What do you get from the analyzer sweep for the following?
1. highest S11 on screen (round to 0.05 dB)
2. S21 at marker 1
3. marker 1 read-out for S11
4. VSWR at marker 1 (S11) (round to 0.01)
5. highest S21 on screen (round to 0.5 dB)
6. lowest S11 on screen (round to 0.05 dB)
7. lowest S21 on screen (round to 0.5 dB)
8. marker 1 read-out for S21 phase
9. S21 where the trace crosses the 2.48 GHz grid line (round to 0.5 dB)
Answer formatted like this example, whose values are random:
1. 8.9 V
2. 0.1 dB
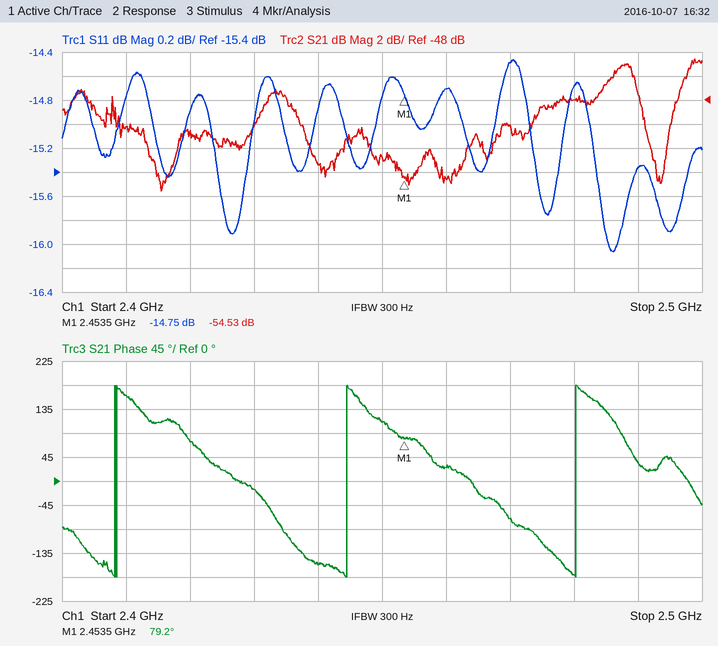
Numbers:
1. -14.45 dB
2. -54.53 dB
3. -14.75 dB
4. 1.45
5. -44.5 dB
6. -16.05 dB
7. -55.5 dB
8. 79.2°
9. -48.0 dB
